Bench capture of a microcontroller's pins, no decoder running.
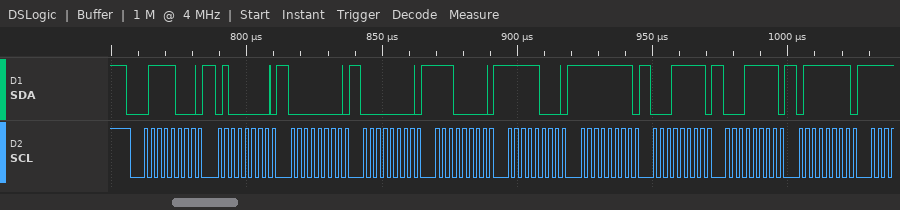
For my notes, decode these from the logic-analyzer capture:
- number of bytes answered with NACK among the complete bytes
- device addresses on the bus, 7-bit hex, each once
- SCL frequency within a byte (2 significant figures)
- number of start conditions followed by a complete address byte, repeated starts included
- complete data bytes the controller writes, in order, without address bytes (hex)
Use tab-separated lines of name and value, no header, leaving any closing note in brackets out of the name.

number of bytes answered with NACK among the complete bytes	0
device addresses on the bus, 7-bit hex, each once	0x3C
SCL frequency within a byte	400 kHz
number of start conditions followed by a complete address byte, repeated starts included	1
complete data bytes the controller writes, in order, without address bytes	40 00 00 E0 F8 FF 1F 1F 7F
